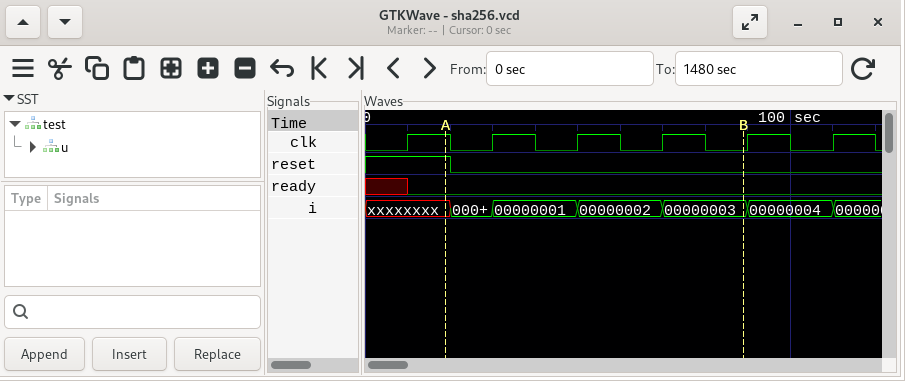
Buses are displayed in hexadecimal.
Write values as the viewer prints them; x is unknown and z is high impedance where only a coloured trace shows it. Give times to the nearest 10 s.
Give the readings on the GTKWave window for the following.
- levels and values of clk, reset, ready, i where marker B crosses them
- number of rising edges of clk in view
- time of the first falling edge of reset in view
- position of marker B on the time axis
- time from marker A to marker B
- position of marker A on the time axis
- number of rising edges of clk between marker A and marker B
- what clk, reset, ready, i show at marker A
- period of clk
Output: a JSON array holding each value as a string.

["clk=0, reset=0, ready=0, i=00000003", "6", "20 s", "90 s", "70 s", "20 s", "3", "clk=1, reset=1, ready=0, i=xxxxxxxx", "20 s"]
